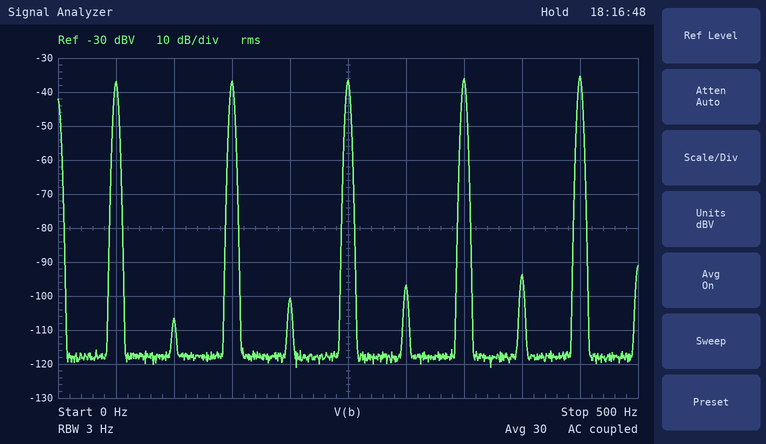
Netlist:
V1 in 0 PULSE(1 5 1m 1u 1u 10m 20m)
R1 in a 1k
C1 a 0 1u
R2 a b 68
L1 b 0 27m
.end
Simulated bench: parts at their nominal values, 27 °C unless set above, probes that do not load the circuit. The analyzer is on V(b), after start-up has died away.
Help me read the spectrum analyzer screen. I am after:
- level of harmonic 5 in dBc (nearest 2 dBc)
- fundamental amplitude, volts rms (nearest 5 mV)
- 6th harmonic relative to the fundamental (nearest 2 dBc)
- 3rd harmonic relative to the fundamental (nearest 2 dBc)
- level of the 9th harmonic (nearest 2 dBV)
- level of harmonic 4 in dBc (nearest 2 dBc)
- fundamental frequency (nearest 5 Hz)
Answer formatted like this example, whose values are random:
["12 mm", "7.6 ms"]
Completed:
["0 dBc", "15 mV", "-60 dBc", "0 dBc", "-36 dBV", "-64 dBc", "50 Hz"]
